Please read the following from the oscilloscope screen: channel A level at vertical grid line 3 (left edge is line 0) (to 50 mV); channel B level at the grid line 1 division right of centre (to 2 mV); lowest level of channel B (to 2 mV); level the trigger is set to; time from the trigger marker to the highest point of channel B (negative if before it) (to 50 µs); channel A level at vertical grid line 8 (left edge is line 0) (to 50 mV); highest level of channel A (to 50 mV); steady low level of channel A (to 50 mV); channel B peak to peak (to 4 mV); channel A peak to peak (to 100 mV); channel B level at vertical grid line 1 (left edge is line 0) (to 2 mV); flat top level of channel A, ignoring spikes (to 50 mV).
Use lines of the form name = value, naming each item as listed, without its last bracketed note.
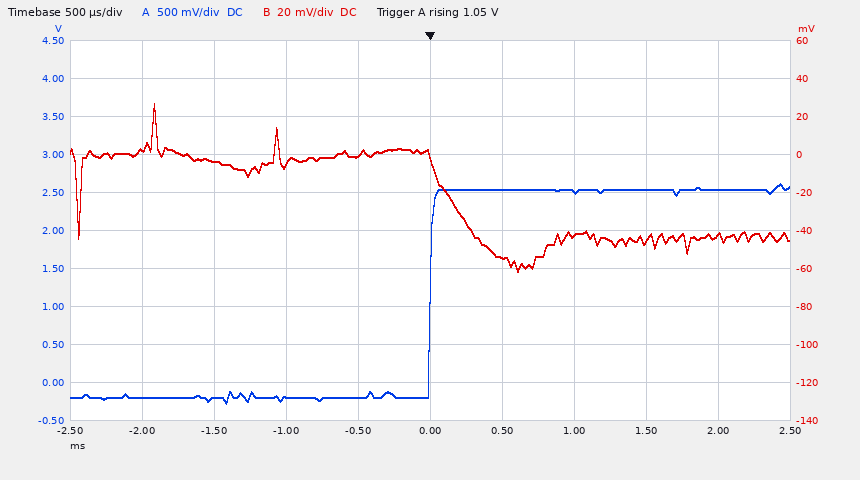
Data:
channel A level at vertical grid line 3 (left edge is line 0) = -200 mV
channel B level at the grid line 1 division right of centre = -54 mV
lowest level of channel B = -62 mV
level the trigger is set to = 1.05 V
time from the trigger marker to the highest point of channel B (negative if before it) = -1.90 ms
channel A level at vertical grid line 8 (left edge is line 0) = 2.55 V
highest level of channel A = 2.60 V
steady low level of channel A = -200 mV
channel B peak to peak = 88 mV
channel A peak to peak = 2.90 V
channel B level at vertical grid line 1 (left edge is line 0) = 2 mV
flat top level of channel A, ignoring spikes = 2.55 V
